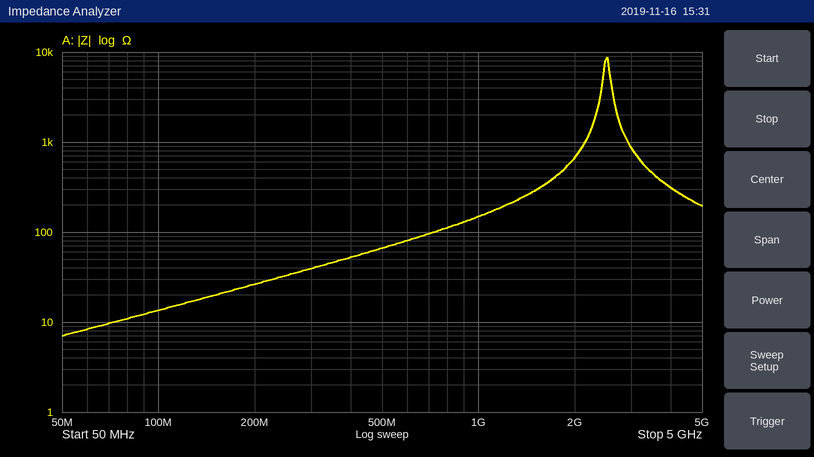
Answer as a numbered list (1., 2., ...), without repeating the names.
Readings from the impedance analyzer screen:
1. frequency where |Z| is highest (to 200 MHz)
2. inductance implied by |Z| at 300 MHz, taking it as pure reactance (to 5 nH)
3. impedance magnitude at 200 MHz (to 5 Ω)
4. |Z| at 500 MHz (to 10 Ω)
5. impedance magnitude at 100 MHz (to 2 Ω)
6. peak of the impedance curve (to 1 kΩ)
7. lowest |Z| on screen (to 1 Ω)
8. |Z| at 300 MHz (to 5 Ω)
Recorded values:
1. 2.6 GHz
2. 20 nH
3. 25 Ω
4. 70 Ω
5. 14 Ω
6. 9 kΩ
7. 7 Ω
8. 40 Ω
